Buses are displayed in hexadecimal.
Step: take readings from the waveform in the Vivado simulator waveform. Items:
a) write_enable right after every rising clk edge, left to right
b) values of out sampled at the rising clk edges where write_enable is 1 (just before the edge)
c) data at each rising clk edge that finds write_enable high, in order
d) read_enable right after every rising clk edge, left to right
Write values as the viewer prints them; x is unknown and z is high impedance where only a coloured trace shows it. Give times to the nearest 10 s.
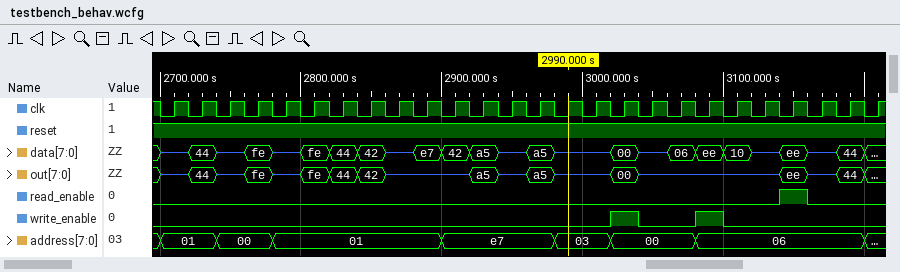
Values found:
0 0 0 0 0 0 0 0 0 0 0 0 0 0 0 0 1 0 0 1 0 0 0 0 0 0
00, z
00, ee
0 0 0 0 0 0 0 0 0 0 0 0 0 0 0 0 0 0 0 0 0 0 1 0 0 0
